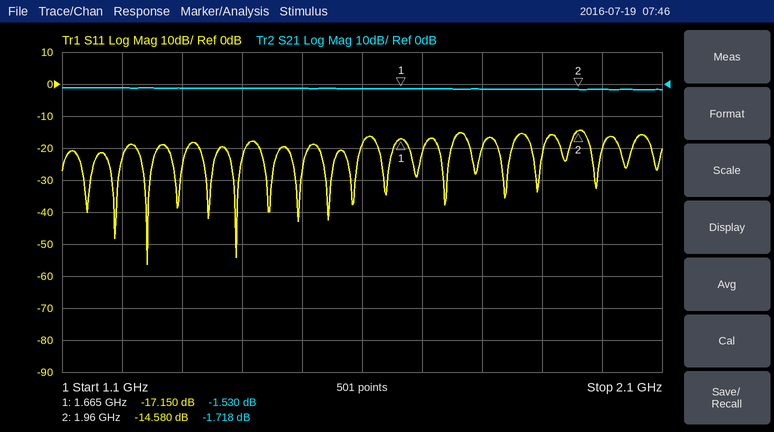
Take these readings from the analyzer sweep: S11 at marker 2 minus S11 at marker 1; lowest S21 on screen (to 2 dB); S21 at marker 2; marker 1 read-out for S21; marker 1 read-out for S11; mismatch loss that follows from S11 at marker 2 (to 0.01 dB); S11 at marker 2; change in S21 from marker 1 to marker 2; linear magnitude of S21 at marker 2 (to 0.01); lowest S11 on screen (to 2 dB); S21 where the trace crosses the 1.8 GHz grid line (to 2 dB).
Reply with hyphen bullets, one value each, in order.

- 2.570 dB
- -2 dB
- -1.718 dB
- -1.530 dB
- -17.150 dB
- 0.15 dB
- -14.580 dB
- -0.188 dB
- 0.82
- -56 dB
- -2 dB
